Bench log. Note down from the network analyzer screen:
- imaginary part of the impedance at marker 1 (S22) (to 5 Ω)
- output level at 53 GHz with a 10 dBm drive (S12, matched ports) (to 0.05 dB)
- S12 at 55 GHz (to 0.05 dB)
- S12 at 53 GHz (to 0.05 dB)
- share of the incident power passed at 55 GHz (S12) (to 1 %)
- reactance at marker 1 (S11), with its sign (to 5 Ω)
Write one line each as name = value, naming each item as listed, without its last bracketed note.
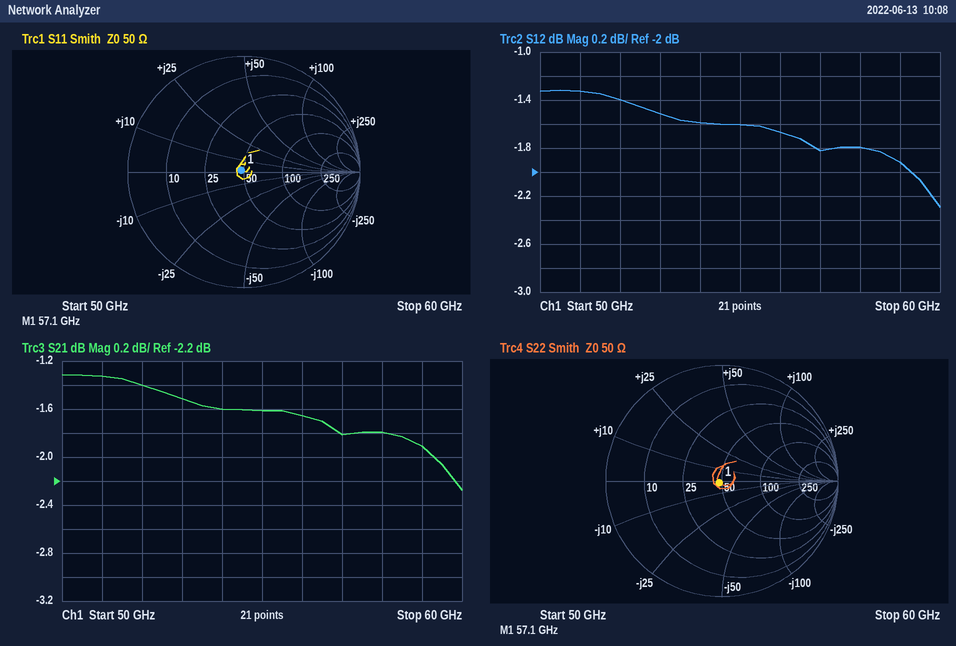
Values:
imaginary part of the impedance at marker 1 (S22) = 0 Ω
output level at 53 GHz with a 10 dBm drive (S12, matched ports) = 8.50 dBm
S12 at 55 GHz = -1.60 dB
S12 at 53 GHz = -1.50 dB
share of the incident power passed at 55 GHz (S12) = 69 %
reactance at marker 1 (S11), with its sign = 0 Ω
